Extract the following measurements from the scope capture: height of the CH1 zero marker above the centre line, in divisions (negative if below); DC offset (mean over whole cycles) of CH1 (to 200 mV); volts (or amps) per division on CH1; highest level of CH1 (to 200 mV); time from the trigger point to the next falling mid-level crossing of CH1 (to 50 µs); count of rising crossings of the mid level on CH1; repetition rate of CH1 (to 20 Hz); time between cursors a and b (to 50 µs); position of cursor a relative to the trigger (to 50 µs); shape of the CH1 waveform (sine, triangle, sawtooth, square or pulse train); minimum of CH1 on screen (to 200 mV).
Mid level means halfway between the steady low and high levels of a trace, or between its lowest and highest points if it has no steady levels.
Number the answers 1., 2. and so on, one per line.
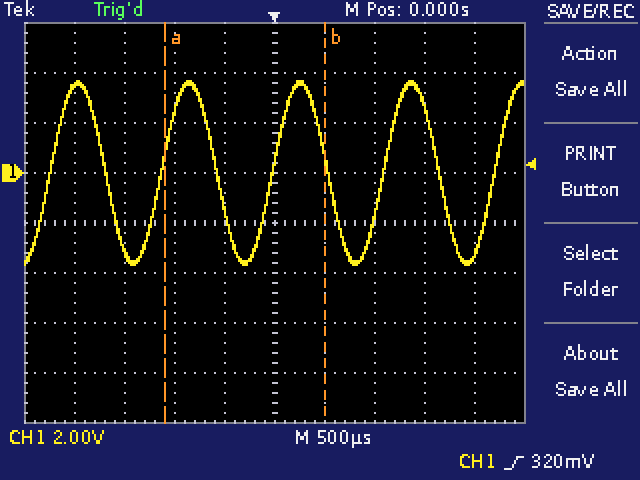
1. +1.0 div
2. 0.0 V
3. 2 V
4. 3.6 V
5. 550 µs
6. 5
7. 900 Hz
8. 1.60 ms
9. -1.10 ms
10. sine
11. -3.6 V
